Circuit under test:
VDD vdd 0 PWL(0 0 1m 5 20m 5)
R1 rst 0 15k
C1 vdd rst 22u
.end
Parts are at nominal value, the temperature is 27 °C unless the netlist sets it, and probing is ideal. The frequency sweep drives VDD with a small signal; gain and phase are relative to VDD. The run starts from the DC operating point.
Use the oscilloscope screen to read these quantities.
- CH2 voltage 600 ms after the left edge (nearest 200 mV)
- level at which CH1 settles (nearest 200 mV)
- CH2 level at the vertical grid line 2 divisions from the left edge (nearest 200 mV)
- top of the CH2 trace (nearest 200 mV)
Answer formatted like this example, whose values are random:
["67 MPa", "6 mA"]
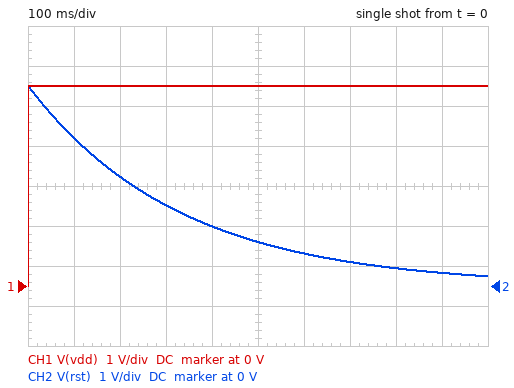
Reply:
["800 mV", "5.0 V", "2.8 V", "5.0 V"]
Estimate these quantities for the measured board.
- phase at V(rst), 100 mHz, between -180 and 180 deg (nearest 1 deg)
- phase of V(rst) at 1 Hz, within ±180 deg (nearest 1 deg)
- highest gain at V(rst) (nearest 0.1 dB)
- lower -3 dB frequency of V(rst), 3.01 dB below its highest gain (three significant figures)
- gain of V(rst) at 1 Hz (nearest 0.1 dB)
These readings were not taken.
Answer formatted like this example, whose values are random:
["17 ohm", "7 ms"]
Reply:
["78 deg", "26 deg", "0 dB", "482 mHz", "-0.9 dB"]
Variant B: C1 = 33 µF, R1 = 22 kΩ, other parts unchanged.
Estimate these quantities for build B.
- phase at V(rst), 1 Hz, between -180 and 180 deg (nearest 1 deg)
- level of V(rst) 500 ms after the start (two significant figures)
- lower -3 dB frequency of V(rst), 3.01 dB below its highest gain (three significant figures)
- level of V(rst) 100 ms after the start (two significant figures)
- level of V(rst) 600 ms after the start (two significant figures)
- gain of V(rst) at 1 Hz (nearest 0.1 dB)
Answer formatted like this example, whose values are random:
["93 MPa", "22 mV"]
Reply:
["12 deg", "2.5 V", "219 mHz", "4.4 V", "2.2 V", "-0.2 dB"]
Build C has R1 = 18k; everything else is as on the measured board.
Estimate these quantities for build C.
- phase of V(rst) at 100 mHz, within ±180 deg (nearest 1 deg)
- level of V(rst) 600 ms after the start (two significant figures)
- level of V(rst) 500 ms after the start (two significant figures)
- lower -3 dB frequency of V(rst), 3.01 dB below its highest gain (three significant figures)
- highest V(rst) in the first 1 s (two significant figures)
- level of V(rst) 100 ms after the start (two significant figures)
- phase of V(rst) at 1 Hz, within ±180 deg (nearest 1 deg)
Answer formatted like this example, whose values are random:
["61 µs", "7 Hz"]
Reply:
["76 deg", "1.1 V", "1.4 V", "402 mHz", "5.0 V", "3.9 V", "22 deg"]
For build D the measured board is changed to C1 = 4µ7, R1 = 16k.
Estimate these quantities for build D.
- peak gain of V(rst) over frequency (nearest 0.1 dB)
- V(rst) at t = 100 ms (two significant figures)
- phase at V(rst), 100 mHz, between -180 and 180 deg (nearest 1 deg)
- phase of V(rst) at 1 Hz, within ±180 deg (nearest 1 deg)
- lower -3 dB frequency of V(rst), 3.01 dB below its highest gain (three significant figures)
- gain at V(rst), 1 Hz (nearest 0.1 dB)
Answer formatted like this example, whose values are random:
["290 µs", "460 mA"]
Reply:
["0 dB", "1.3 V", "87 deg", "65 deg", "2.12 Hz", "-7.4 dB"]
